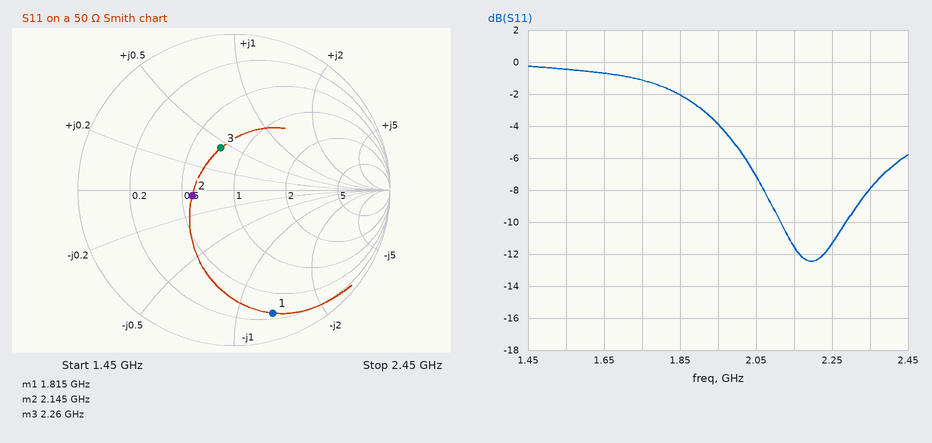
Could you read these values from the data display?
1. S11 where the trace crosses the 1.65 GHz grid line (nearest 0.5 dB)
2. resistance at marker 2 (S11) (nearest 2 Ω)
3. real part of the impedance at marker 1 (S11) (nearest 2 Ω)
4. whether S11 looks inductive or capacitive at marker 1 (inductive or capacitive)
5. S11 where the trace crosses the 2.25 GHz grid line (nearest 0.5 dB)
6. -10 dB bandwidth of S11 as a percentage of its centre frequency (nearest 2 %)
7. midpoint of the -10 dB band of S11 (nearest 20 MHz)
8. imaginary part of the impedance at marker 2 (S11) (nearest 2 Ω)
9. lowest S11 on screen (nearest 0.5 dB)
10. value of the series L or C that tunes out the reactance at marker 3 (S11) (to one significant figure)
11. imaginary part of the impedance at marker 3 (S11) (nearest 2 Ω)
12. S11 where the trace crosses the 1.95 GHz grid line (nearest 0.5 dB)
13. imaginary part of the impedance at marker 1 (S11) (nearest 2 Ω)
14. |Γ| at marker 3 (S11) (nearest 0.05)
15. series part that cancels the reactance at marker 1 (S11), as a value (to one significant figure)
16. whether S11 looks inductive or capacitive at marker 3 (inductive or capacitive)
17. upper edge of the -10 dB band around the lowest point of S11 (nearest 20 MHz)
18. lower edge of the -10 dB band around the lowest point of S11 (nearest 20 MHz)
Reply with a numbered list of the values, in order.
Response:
1. -0.5 dB
2. 28 Ω
3. 14 Ω
4. capacitive
5. -11.5 dB
6. 8 %
7. 2.20 GHz
8. -2 Ω
9. -12.5 dB
10. 3 pF
11. +22 Ω
12. -4.0 dB
13. -66 Ω
14. 0.30
15. 6 nH
16. inductive
17. 2.28 GHz
18. 2.12 GHz
